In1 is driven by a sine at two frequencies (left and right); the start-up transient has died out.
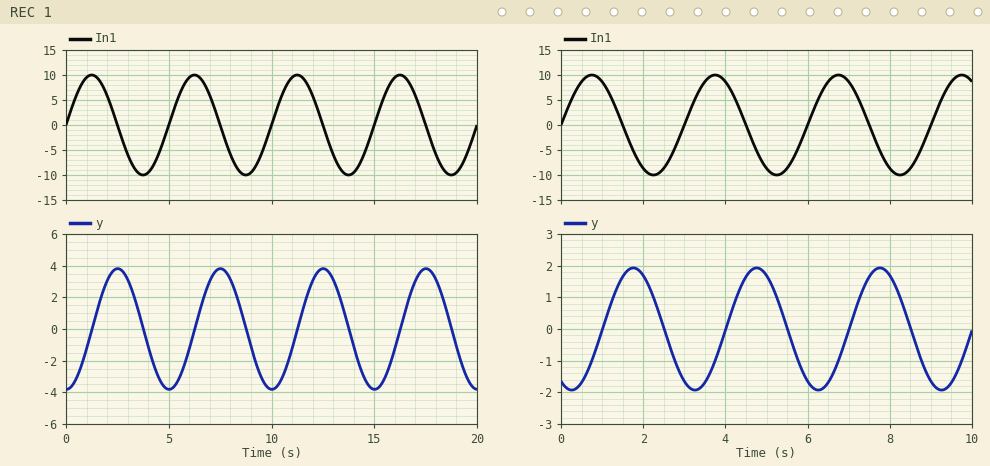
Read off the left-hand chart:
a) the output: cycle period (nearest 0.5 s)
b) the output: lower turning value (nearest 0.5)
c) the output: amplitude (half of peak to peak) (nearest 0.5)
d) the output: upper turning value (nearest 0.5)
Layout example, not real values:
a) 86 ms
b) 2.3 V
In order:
a) 5.0 s
b) -4.0
c) 4.0
d) 4.0
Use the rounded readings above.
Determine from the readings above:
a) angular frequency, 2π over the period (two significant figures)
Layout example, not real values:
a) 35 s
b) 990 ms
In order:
a) 1.3 rad/s
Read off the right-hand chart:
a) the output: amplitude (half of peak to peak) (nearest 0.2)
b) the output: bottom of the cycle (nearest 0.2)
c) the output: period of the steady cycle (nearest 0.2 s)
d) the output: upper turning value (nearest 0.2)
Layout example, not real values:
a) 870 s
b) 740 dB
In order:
a) 2.0
b) -2.0
c) 3.0 s
d) 2.0
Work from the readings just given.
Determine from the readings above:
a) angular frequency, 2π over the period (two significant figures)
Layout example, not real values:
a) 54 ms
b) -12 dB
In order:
a) 2.1 rad/s
